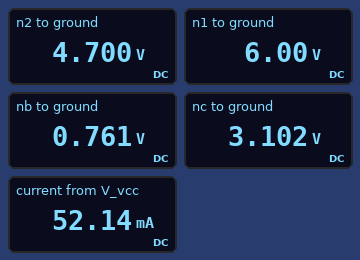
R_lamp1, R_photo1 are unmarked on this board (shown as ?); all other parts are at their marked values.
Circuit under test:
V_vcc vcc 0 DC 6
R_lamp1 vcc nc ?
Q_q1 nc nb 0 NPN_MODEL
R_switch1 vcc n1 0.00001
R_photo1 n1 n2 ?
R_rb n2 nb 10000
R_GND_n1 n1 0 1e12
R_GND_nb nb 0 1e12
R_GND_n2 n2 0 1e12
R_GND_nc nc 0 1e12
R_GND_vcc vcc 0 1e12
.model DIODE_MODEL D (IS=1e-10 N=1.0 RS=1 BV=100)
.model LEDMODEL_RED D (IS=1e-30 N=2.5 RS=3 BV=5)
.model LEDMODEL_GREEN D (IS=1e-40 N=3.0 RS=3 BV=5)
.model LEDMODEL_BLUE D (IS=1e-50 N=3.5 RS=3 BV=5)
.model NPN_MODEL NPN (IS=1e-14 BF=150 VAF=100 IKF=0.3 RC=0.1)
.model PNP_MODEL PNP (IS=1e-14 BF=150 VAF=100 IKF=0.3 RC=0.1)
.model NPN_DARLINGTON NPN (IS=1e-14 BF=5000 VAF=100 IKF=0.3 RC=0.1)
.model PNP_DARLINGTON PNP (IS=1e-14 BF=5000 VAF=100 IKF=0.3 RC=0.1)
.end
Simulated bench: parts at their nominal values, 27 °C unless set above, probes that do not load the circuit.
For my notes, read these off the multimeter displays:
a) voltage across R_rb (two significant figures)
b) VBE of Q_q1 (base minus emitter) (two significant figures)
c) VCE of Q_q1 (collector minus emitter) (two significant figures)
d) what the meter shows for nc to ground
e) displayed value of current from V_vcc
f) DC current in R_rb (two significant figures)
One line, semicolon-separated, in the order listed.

3.9 V; 760 mV; 3.1 V; 3.102 V; 52.14 mA; 390 µA
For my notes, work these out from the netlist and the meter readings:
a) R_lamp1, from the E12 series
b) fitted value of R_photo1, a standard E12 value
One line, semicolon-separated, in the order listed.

56 Ω; 3.3 kΩ
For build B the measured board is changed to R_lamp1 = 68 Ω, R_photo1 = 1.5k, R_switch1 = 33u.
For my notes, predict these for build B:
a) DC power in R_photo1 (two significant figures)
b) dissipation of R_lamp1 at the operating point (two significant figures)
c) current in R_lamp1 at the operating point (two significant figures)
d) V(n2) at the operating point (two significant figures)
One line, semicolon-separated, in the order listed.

310 µW; 230 mW; 58 mA; 5.3 V
